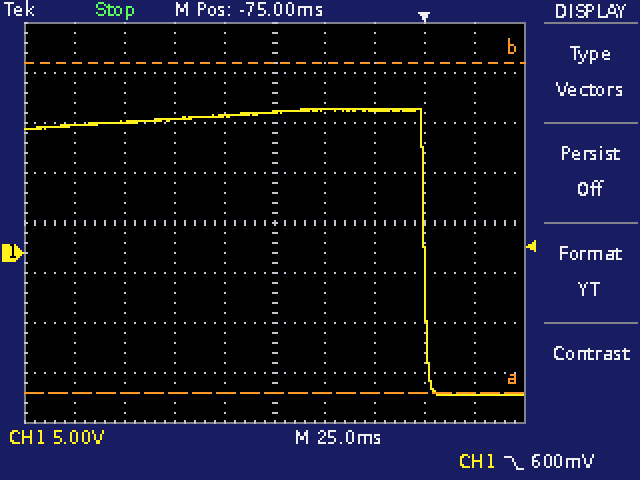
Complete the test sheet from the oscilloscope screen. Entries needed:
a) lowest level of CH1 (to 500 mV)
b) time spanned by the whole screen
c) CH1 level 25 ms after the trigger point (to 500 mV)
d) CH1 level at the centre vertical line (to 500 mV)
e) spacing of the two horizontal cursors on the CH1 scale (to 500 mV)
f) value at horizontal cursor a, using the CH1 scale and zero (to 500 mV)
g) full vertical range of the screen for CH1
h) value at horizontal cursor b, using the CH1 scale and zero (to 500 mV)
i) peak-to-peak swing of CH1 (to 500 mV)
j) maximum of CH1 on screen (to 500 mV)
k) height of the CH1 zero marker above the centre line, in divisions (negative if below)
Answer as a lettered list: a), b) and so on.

a) -14.0 V
b) 250 ms
c) -14.0 V
d) 14.0 V
e) 33.0 V
f) -14.0 V
g) 40 V
h) 19.0 V
i) 28.5 V
j) 14.5 V
k) -0.6 div
